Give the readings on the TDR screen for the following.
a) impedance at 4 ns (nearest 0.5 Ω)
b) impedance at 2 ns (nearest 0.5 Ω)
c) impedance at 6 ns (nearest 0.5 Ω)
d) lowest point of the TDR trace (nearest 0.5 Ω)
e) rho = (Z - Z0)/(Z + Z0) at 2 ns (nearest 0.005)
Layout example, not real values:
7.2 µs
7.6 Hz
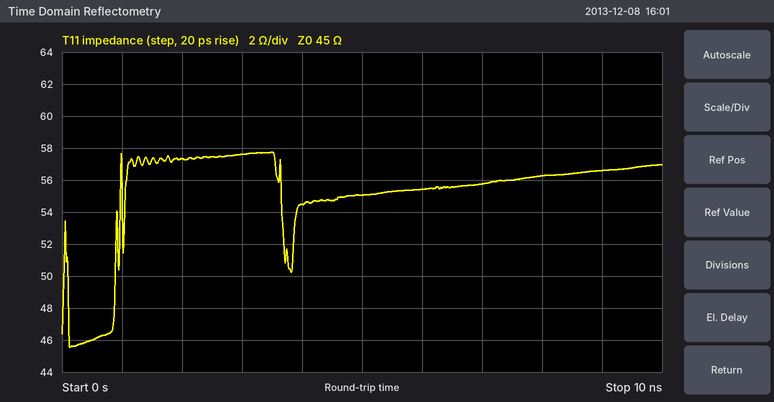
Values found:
54.5 Ω
57.5 Ω
55.5 Ω
45.5 Ω
+0.120
